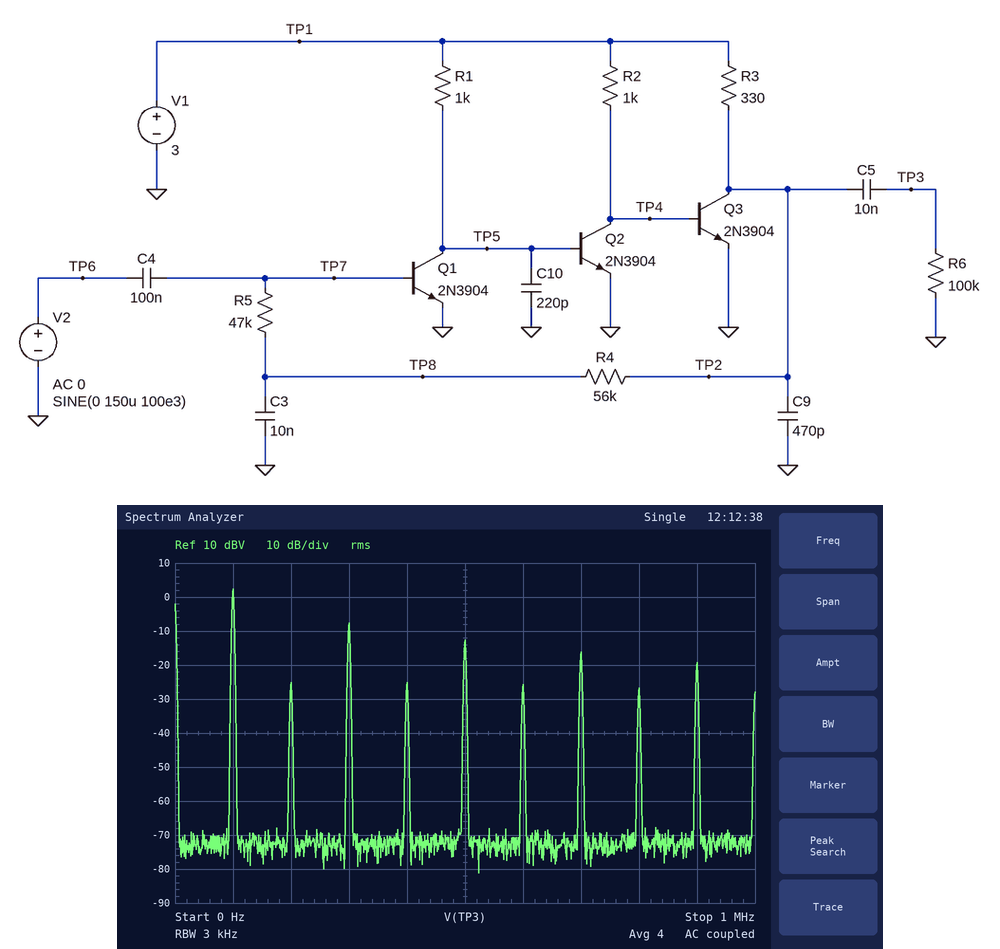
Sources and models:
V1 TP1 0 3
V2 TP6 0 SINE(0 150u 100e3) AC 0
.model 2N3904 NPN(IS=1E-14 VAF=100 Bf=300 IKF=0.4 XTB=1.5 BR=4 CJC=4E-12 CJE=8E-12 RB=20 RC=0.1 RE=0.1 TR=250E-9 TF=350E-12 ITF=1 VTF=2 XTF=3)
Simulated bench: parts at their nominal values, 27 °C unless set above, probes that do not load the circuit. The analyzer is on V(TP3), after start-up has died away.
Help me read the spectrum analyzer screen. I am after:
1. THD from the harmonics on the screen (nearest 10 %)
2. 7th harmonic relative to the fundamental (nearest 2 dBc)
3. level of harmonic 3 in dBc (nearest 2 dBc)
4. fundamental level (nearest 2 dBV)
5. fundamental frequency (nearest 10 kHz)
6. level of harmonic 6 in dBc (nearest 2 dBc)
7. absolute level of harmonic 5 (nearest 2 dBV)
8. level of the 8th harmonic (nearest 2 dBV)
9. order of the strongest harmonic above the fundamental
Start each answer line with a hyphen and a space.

- 40 %
- -18 dBc
- -10 dBc
- 2 dBV
- 100 kHz
- -28 dBc
- -12 dBV
- -26 dBV
- 3
